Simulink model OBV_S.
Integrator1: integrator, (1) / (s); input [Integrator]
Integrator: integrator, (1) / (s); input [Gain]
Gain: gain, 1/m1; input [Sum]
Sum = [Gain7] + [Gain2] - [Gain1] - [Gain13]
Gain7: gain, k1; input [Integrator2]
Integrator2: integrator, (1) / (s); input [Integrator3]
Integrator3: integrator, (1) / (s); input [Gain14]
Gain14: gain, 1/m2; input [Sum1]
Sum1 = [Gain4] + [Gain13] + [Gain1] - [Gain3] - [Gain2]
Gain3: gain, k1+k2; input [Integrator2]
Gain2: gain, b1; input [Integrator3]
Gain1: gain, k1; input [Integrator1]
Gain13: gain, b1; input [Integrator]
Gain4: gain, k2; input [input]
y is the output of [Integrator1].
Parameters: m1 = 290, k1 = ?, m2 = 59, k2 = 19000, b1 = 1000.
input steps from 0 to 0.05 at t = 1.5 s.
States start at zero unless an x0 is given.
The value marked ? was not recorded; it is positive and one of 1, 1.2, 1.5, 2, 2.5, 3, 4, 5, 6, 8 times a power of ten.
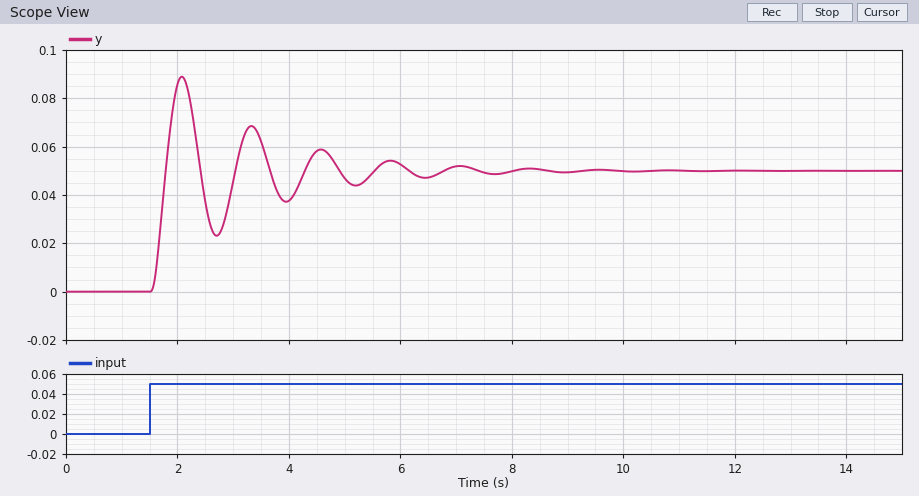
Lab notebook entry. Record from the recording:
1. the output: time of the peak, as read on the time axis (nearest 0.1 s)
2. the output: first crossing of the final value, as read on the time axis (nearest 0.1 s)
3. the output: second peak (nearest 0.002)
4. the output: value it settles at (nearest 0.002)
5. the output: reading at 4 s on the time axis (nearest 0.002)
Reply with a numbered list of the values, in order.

1. 2.1 s
2. 1.8 s
3. 0.068
4. 0.050
5. 0.038
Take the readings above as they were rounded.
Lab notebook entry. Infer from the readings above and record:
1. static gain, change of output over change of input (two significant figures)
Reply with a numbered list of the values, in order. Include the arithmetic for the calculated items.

1. (0.05 - 0) / (0.05 - 0) = 1.0
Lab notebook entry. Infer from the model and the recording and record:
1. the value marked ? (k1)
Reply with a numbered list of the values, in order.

1. 12000
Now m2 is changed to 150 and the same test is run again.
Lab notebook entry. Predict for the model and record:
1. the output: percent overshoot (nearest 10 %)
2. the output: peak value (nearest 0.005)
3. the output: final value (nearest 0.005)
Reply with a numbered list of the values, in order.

1. 90 %
2. 0.095
3. 0.050
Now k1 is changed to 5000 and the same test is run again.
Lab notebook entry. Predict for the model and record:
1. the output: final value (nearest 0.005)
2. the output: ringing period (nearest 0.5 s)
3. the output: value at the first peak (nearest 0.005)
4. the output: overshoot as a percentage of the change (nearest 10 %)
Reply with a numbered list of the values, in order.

1. 0.050
2. 1.5 s
3. 0.075
4. 50 %
